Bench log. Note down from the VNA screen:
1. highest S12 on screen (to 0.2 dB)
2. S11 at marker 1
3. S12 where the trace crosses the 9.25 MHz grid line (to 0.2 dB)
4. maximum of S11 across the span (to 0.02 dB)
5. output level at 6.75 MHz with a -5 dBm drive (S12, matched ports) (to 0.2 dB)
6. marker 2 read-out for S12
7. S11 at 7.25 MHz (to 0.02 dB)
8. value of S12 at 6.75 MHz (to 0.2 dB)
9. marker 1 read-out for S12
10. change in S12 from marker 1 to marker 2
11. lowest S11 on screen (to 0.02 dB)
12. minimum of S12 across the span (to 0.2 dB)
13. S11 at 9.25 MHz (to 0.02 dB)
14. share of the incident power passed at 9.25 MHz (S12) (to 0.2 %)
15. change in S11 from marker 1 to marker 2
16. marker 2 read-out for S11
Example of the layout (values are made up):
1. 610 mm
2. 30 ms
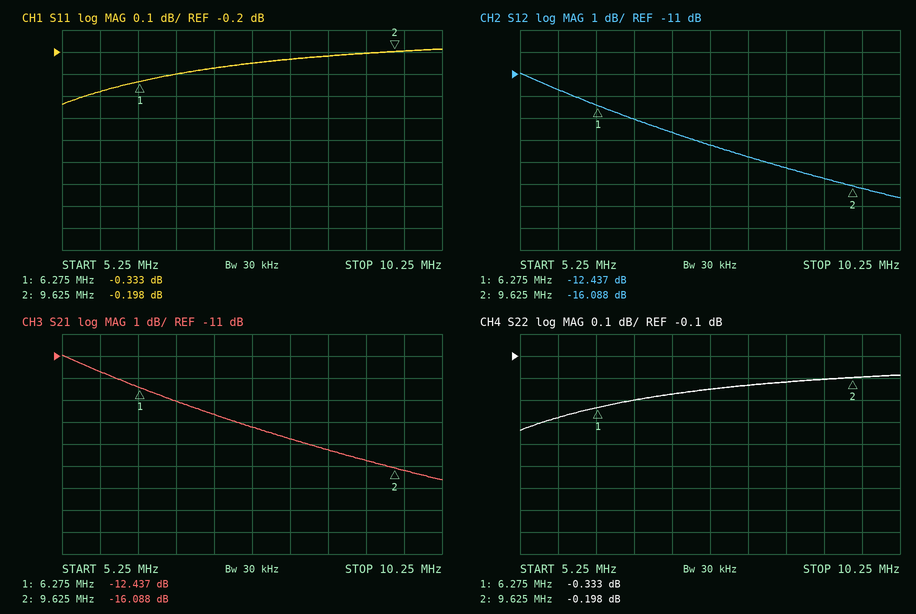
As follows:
1. -11.0 dB
2. -0.333 dB
3. -15.8 dB
4. -0.18 dB
5. -18.0 dBm
6. -16.088 dB
7. -0.28 dB
8. -13.0 dB
9. -12.437 dB
10. -3.651 dB
11. -0.44 dB
12. -16.6 dB
13. -0.20 dB
14. 2.6 %
15. 0.135 dB
16. -0.198 dB
